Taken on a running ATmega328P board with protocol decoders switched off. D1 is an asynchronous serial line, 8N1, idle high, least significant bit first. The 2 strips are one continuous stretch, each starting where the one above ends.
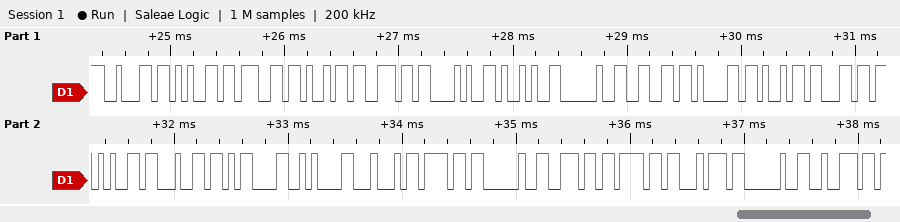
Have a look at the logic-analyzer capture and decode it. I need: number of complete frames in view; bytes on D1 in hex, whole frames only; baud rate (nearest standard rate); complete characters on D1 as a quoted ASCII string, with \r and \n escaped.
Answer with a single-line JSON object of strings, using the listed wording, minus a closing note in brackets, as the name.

{"number of complete frames in view": "24", "bytes on D1 in hex, whole frames only": "0x62 0x65 0x67 0x69 0x6E 0x28 0x29 0x20 0x66 0x61 0x69 0x6C 0x65 0x64 0x0D 0x0A 0x44 0x6F 0x20 0x6E 0x6F 0x74 0x20 0x72", "baud rate": "19200 baud", "complete characters on D1 as a quoted ASCII string, with \\r and \\n escaped": "\"begin() failed\\r\\nDo not r\""}
